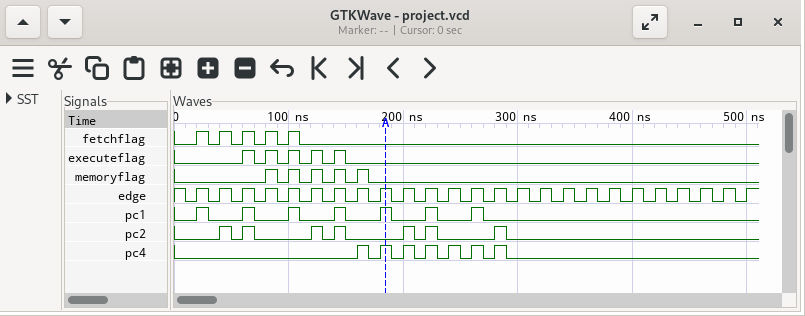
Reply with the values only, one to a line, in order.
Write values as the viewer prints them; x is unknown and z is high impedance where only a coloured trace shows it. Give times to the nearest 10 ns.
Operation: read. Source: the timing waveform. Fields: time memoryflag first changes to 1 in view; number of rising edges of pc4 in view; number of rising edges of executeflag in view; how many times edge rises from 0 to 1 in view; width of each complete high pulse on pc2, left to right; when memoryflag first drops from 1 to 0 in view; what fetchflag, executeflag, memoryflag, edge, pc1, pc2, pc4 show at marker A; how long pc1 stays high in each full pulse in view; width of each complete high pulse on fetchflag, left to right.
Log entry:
80 ns
7
5
25
10 ns, 10 ns, 10 ns, 10 ns, 10 ns, 10 ns, 10 ns
90 ns
fetchflag=0, executeflag=0, memoryflag=0, edge=1, pc1=1, pc2=0, pc4=1
10 ns, 10 ns, 10 ns, 10 ns, 10 ns, 10 ns, 10 ns
10 ns, 10 ns, 10 ns, 10 ns, 10 ns
